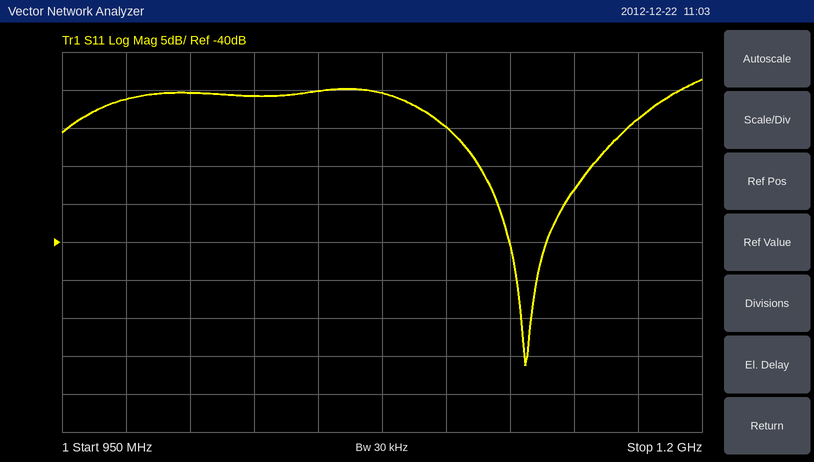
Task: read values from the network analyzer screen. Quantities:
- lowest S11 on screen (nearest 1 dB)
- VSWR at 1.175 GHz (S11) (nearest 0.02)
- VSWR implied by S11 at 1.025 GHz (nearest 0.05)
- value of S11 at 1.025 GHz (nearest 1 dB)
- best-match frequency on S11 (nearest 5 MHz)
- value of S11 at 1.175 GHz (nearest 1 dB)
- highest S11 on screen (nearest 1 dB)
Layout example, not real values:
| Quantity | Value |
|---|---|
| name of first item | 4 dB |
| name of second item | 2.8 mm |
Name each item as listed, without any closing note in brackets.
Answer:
| Quantity | Value |
|---|---|
| lowest S11 on screen | -56 dB |
| VSWR at 1.175 GHz (S11) | 1.14 |
| VSWR implied by S11 at 1.025 GHz | 1.20 |
| value of S11 at 1.025 GHz | -21 dB |
| best-match frequency on S11 | 1.130 GHz |
| value of S11 at 1.175 GHz | -24 dB |
| highest S11 on screen | -19 dB |
